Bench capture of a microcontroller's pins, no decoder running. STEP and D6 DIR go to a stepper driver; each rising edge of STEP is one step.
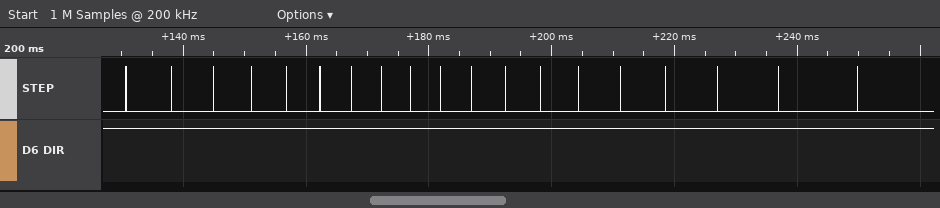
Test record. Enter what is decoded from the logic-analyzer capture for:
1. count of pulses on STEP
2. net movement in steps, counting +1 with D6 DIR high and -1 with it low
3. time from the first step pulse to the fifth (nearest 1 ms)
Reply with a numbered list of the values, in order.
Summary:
1. 19
2. +19
3. 26 ms
